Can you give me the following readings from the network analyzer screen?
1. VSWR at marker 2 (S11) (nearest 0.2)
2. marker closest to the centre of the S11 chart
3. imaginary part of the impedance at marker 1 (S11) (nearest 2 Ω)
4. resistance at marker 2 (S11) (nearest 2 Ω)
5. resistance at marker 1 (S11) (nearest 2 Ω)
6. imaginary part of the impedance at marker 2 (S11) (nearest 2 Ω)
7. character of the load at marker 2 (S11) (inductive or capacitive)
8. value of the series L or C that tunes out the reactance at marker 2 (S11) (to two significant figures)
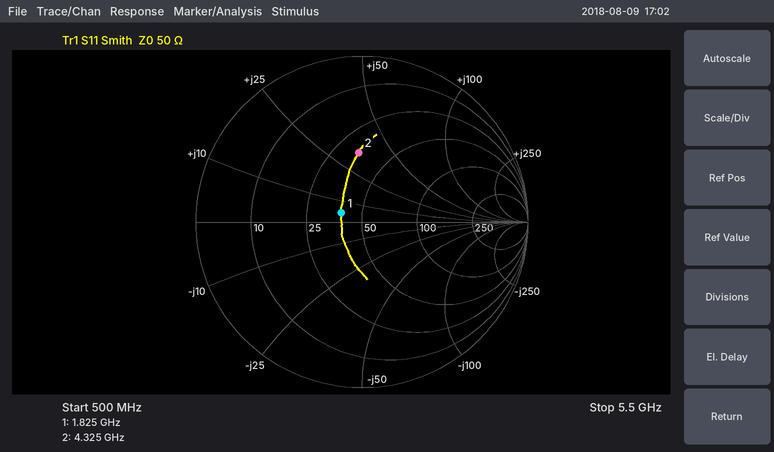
2.4
marker 1
+4 Ω
34 Ω
38 Ω
+34 Ω
inductive
1.1 pF
